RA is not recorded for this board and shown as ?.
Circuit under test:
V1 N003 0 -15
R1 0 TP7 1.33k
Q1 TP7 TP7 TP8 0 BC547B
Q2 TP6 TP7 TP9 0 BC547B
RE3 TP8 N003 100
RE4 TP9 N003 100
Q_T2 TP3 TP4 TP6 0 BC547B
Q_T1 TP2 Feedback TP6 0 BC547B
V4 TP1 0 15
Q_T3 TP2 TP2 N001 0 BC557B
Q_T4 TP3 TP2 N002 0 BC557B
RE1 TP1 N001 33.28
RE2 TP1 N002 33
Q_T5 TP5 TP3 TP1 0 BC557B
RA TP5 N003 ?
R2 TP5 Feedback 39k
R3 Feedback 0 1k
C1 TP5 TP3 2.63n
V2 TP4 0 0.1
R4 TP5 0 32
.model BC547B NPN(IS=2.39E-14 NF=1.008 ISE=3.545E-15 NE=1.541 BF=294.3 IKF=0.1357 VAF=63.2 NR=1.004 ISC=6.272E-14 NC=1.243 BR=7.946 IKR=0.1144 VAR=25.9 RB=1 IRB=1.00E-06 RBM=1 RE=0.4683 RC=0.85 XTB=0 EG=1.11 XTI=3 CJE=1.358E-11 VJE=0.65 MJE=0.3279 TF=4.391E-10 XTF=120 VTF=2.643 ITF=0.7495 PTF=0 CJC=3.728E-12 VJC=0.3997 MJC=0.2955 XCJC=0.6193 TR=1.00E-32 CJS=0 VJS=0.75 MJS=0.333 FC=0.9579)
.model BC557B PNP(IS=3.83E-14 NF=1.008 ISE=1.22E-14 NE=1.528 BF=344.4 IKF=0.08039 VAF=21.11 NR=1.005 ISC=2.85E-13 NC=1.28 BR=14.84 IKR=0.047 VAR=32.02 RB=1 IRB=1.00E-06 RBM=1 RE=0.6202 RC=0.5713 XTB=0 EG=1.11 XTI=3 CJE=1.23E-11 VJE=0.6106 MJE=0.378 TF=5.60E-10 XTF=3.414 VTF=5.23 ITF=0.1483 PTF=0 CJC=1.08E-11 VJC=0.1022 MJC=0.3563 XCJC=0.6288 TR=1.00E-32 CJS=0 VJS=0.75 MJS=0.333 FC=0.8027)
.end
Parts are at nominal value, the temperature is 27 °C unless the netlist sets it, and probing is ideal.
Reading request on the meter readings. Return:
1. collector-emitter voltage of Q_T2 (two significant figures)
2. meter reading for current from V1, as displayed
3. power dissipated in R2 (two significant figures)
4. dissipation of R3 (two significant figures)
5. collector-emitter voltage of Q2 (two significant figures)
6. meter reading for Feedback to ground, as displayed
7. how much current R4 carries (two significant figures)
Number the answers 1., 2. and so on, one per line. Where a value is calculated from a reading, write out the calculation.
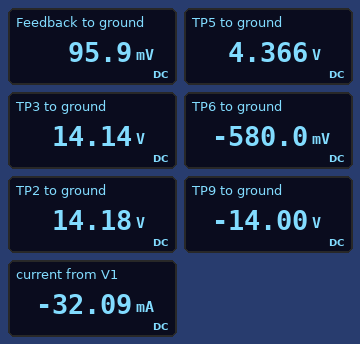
1. 14.14 V - (-580 mV) = 15 V
2. -32.09 mA
3. (4.366 V - 95.9 mV)^2 / 39 kΩ = 470 µW
4. (95.9 mV)^2 / 1 kΩ = 9.2 µW
5. -580 mV - (-14 V) = 13 V
6. 95.9 mV
7. (4.366 V) / 32 Ω = 140 mA
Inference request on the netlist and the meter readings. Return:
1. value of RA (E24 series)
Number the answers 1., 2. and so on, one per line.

1. 1.6 kΩ
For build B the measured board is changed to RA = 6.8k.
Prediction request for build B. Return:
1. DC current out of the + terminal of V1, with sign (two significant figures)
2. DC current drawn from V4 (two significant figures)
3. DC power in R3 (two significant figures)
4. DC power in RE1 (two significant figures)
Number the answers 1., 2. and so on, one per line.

1. -23 mA
2. 150 mA
3. 9.3 µW
4. 720 µW
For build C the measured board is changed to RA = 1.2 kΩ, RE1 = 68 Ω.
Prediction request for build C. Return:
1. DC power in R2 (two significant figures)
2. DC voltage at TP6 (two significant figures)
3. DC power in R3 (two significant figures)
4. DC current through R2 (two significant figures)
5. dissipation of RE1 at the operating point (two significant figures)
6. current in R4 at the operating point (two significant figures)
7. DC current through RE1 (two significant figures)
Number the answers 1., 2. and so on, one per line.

1. 310 µW
2. -590 mV
3. 6.3 µW
4. 89 µA
5. 730 µW
6. 110 mA
7. 3.3 mA
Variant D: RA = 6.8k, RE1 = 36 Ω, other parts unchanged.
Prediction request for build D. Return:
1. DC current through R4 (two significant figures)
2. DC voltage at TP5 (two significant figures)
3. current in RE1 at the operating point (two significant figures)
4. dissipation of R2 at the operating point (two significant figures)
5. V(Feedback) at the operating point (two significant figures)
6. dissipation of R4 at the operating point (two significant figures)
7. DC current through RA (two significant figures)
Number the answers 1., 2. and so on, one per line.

1. 130 mA
2. 4.3 V
3. 4.5 mA
4. 450 µW
5. 95 mV
6. 580 mW
7. 2.8 mA
